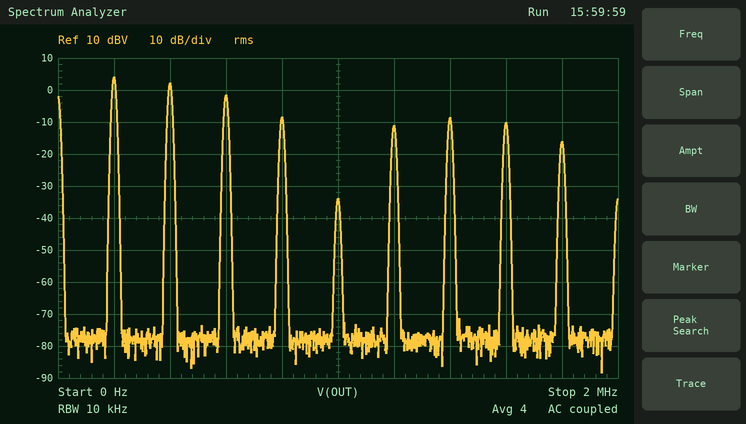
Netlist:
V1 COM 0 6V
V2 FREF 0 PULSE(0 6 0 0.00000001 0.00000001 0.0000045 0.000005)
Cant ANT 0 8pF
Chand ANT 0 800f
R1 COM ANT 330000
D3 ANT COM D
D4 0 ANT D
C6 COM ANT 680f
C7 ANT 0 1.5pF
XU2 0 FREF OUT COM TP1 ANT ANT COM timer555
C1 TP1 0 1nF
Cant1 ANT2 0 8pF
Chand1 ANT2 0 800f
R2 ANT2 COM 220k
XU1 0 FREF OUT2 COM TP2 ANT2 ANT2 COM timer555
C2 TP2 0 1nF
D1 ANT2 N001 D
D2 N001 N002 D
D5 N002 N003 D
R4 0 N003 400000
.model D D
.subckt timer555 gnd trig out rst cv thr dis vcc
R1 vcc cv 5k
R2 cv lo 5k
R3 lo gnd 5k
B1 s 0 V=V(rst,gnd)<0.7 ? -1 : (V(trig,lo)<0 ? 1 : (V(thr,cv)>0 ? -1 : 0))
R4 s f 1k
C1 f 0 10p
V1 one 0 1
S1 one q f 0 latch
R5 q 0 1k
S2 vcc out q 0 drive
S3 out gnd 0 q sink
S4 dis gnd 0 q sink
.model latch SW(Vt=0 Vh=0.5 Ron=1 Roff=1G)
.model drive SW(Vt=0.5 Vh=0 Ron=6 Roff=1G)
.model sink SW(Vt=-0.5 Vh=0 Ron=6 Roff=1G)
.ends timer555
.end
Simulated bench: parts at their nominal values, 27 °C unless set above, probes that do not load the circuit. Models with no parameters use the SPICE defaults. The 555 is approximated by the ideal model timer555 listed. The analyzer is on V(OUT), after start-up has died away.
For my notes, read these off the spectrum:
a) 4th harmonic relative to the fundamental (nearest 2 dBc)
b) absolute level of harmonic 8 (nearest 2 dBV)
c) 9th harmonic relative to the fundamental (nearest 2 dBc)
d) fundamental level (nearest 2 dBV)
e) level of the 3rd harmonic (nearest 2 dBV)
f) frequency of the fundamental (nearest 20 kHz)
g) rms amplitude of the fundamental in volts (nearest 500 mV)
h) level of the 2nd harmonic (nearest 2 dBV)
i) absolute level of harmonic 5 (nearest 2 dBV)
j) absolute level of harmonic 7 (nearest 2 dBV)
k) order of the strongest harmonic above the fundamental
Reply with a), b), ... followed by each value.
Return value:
a) -12 dBc
b) -10 dBV
c) -20 dBc
d) 4 dBV
e) -2 dBV
f) 200 kHz
g) 1.5 V
h) 2 dBV
i) -34 dBV
j) -8 dBV
k) 2
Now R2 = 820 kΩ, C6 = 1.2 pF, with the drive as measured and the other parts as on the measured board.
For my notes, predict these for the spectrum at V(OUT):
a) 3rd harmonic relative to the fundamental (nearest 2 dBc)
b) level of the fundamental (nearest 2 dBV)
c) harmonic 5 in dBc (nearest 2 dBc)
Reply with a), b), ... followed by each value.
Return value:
a) -4 dBc
b) 2 dBV
c) -14 dBc
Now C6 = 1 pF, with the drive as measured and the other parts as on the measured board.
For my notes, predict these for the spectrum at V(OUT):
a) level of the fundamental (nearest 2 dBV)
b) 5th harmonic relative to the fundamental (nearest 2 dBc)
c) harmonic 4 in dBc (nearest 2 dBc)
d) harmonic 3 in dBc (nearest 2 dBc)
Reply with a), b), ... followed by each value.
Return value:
a) 4 dBV
b) -18 dBc
c) -8 dBc
d) -4 dBc
